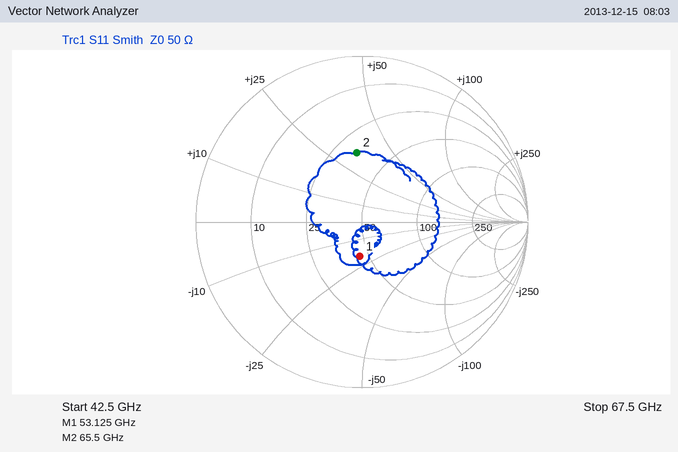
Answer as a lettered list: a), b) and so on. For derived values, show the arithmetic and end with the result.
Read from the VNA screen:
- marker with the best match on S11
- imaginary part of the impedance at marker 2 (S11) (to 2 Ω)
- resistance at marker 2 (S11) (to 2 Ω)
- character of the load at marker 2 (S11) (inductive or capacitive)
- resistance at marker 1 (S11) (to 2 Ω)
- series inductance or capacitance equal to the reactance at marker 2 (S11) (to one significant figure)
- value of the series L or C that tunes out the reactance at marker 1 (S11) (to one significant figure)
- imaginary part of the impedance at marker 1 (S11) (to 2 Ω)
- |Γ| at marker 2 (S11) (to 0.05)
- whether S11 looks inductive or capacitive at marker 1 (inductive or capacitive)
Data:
a) marker 1
b) +34 Ω
c) 34 Ω
d) inductive
e) 44 Ω
f) L = 34 Ω/(2π × 65.5 GHz) ≈ 82.6 pH, so 80 pH to one significant figure
g) L = 20 Ω/(2π × 53.125 GHz) ≈ 60 pH
h) -20 Ω
i) 0.40
j) capacitive
